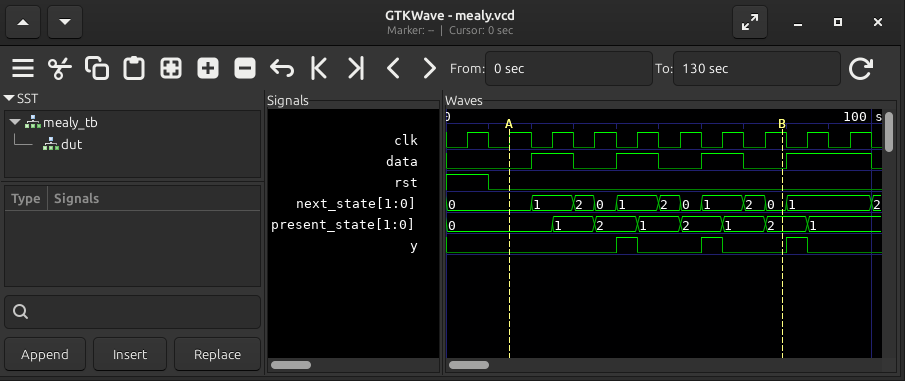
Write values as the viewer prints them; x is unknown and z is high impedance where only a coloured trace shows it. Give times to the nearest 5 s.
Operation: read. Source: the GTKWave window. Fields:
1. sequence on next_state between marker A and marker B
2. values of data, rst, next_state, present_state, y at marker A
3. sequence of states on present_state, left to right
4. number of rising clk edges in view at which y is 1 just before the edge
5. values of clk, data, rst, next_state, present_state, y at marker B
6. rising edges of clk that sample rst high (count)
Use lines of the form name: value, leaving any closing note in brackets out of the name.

sequence on next_state between marker A and marker B: 0, 1, 2, 0, 1, 2, 0, 1, 2, 0
values of data, rst, next_state, present_state, y at marker A: data=0, rst=0, next_state=0, present_state=0, y=0
sequence of states on present_state, left to right: 0, 1, 2, 1, 2, 1, 2, 1
number of rising clk edges in view at which y is 1 just before the edge: 3
values of clk, data, rst, next_state, present_state, y at marker B: clk=1, data=0, rst=0, next_state=0, present_state=2, y=0
rising edges of clk that sample rst high: 1
